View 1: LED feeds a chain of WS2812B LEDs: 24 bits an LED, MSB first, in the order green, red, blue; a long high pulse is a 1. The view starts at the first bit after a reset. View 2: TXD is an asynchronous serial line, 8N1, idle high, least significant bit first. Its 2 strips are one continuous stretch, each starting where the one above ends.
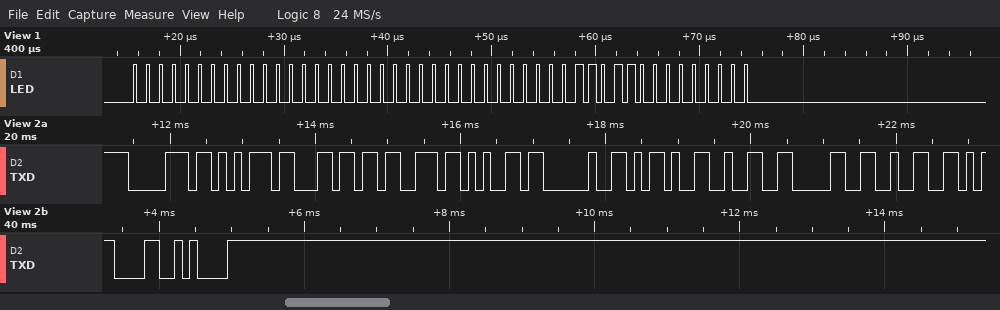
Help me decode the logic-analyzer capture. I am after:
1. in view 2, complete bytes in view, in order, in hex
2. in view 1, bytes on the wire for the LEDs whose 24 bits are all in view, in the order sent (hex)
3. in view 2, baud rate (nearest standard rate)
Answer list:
0x70 0x75 0x6C 0x73 0x65 0x20 0x2D 0x32 0x30 0x32 0x0D 0x0A
00 00 00 00 36 00
9600 baud
